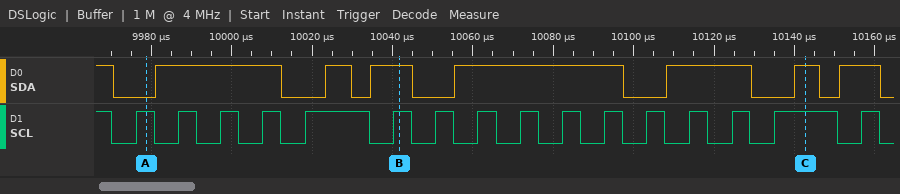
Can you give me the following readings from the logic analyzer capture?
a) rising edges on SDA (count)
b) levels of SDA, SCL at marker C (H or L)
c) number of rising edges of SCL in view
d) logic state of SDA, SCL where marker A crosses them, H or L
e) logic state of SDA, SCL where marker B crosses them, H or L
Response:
7
SDA=H, SCL=H
16
SDA=L, SCL=H
SDA=H, SCL=H
